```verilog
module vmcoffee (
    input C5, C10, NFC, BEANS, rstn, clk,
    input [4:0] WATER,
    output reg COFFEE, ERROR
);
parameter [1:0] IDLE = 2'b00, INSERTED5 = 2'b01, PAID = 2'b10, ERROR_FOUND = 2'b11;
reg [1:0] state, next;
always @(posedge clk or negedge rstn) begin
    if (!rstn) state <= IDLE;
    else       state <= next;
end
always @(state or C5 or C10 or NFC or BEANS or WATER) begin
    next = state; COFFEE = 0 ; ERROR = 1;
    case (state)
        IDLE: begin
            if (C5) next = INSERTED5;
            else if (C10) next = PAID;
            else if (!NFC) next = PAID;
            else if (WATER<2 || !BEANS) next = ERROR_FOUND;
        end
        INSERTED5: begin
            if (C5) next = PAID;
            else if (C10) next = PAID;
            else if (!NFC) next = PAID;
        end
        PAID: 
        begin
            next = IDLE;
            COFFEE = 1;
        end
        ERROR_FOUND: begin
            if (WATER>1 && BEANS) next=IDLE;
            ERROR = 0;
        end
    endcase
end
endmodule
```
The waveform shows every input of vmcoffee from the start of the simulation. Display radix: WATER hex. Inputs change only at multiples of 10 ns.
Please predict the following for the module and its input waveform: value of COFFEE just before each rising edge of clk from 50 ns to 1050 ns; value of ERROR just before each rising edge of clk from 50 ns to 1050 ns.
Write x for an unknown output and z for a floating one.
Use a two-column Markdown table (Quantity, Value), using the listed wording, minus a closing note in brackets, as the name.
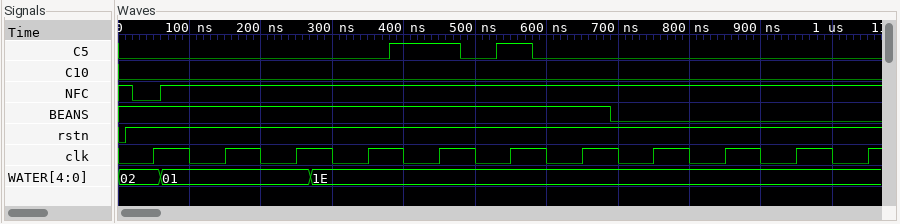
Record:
| Quantity | Value |
|---|---|
| value of COFFEE just before each rising edge of clk from 50 ns to 1050 ns | 0 1 0 0 0 0 1 0 0 0 0 |
| value of ERROR just before each rising edge of clk from 50 ns to 1050 ns | 1 1 1 0 1 1 1 1 0 0 0 |
